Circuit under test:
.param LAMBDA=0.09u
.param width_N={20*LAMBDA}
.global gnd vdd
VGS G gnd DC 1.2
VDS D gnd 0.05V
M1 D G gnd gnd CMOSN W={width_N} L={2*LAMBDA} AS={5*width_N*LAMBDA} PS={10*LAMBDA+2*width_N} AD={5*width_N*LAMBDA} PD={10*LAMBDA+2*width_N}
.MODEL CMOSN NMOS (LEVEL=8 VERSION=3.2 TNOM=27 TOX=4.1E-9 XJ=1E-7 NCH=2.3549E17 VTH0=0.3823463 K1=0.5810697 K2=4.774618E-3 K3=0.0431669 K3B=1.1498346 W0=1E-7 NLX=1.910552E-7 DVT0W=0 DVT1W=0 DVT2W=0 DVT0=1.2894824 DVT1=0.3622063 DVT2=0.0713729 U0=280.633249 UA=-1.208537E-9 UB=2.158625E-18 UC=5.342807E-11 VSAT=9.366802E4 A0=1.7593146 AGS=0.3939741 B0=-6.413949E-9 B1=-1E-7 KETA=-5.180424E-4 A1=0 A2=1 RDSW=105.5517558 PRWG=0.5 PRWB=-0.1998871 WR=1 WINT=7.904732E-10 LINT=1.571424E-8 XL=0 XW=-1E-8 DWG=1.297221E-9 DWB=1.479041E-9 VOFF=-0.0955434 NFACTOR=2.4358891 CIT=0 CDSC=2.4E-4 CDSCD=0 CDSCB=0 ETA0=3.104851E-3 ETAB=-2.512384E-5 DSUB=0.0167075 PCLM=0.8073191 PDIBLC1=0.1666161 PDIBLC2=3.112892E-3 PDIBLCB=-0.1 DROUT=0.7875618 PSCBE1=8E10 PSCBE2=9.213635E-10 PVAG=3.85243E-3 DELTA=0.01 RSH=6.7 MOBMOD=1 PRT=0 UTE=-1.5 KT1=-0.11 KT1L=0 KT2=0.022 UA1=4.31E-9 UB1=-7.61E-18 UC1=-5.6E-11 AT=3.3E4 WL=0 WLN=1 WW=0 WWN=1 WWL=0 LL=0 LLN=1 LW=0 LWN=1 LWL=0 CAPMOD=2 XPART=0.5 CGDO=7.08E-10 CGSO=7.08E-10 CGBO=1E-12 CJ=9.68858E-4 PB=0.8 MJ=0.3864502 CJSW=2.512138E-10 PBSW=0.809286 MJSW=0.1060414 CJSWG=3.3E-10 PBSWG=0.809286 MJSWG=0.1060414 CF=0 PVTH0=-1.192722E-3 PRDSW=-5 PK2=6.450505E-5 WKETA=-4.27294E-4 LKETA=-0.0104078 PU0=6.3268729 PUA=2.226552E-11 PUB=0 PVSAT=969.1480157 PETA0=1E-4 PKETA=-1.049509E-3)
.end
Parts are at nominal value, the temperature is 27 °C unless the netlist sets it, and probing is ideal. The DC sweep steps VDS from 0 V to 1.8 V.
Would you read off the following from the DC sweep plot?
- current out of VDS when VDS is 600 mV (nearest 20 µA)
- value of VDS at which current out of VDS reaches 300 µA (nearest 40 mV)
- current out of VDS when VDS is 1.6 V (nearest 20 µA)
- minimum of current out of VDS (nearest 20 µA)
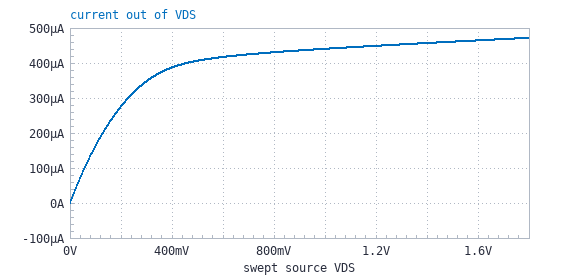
420 µA
240 mV
460 µA
0 A
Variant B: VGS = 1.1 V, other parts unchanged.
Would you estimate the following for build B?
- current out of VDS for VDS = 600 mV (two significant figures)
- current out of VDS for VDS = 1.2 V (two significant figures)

340 µA
360 µA
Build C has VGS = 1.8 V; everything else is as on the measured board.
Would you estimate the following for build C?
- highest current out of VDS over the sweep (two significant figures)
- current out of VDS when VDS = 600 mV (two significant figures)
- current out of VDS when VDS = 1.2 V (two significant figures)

1.0 mA
880 µA
970 µA
